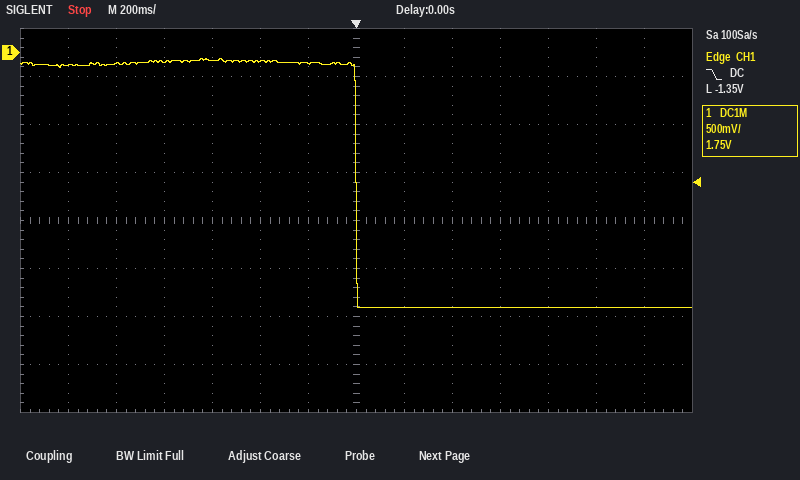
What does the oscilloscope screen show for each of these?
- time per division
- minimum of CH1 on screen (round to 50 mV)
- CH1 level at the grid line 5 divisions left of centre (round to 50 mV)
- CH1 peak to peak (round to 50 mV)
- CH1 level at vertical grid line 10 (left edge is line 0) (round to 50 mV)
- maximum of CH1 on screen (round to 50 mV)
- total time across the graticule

200 ms
-2.65 V
-100 mV
2.60 V
-2.65 V
-50 mV
2.8 s
